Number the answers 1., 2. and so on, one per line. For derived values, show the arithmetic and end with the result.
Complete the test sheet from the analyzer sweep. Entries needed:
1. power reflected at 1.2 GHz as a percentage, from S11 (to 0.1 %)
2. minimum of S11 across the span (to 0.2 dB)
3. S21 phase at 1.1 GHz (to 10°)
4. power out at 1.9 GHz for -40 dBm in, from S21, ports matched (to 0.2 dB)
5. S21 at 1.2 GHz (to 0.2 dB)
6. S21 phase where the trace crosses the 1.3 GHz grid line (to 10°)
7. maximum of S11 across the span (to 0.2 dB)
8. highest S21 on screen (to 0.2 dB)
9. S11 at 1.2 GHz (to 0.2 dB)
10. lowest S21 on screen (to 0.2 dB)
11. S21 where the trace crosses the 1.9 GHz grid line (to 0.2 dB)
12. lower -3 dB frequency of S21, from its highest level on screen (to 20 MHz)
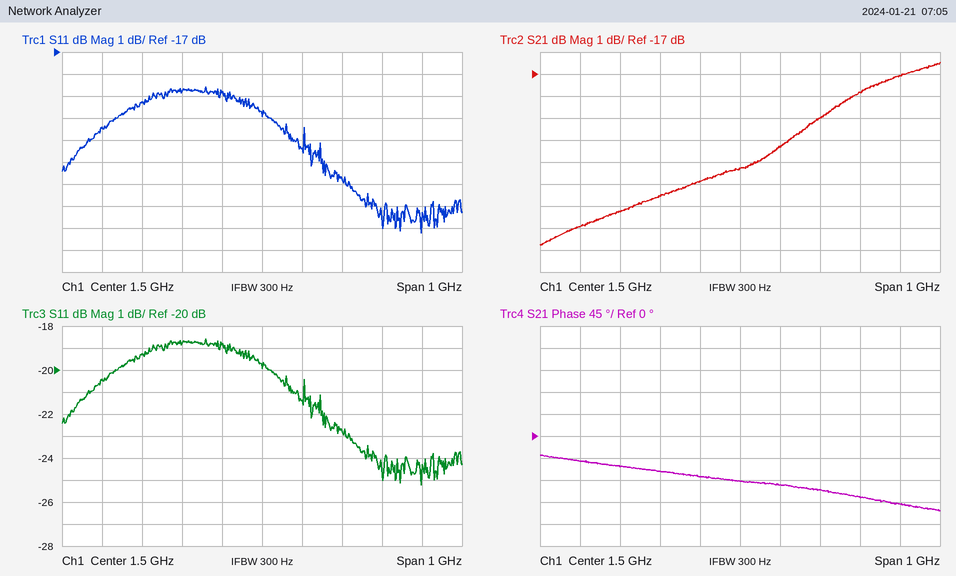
1. 10^(-19.2/10) ≈ 1.2 %
2. -25.2 dB
3. -50°
4. -40 dBm + (-17.0 dB) = -57.0 dBm
5. -23.2 dB
6. -70°
7. -18.6 dB
8. -16.4 dB
9. -19.2 dB
10. -24.8 dB
11. -17.0 dB
12. 1.66 GHz
